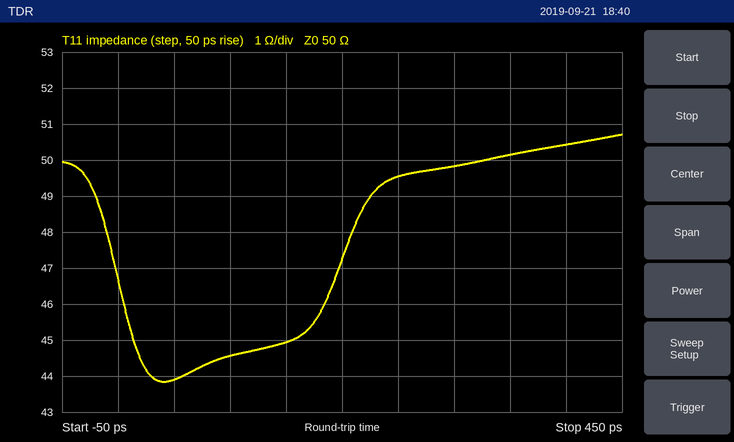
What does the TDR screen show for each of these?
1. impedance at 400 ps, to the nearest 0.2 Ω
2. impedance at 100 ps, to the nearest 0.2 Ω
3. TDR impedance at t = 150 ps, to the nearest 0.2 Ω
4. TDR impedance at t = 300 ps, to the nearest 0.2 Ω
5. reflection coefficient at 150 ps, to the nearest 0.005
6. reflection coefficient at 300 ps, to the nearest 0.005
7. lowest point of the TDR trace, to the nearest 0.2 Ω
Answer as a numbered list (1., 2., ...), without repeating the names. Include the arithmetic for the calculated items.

1. 50.4 Ω
2. 44.6 Ω
3. 45.0 Ω
4. 49.8 Ω
5. (45 − 50)/(45 + 50) ≈ -0.0526, so -0.055 to the nearest 0.005
6. (49.8 − 50)/(49.8 + 50) ≈ 0.000
7. 43.8 Ω
